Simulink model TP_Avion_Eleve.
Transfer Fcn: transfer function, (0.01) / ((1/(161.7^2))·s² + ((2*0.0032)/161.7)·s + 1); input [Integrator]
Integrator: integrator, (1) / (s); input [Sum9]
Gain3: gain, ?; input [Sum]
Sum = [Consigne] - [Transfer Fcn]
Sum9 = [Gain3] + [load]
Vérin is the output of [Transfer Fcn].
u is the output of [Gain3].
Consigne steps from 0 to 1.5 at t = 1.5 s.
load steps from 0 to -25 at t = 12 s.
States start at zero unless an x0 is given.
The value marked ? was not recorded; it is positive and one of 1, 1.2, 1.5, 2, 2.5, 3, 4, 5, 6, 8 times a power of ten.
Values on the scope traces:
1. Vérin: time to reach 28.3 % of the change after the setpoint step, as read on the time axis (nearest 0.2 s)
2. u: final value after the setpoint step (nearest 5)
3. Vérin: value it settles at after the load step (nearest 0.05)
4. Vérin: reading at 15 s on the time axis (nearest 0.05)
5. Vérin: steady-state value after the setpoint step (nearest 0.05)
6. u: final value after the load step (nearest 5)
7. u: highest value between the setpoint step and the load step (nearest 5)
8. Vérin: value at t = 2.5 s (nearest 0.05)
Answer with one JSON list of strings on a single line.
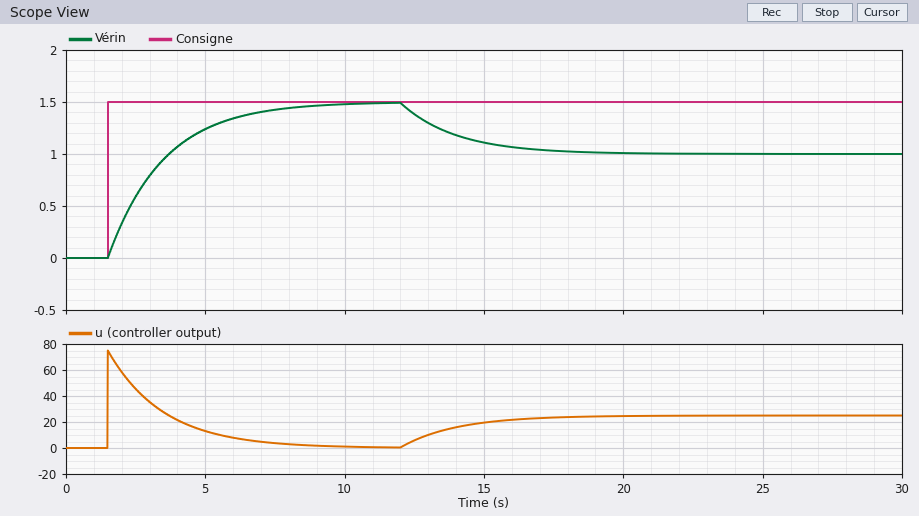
["2.2 s", "0", "1.00", "1.10", "1.50", "25", "75", "0.60"]
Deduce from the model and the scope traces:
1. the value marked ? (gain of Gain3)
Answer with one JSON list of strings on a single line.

["50"]
